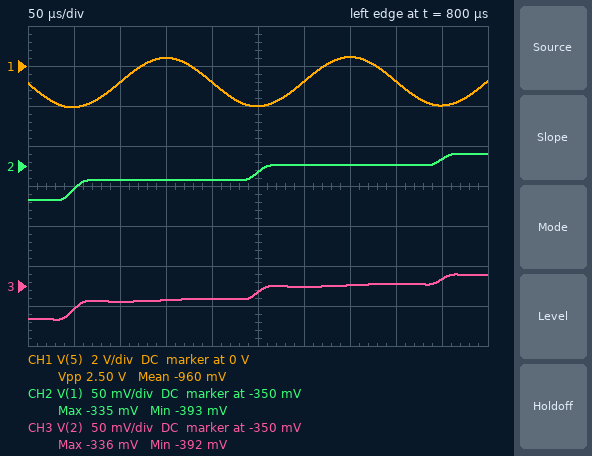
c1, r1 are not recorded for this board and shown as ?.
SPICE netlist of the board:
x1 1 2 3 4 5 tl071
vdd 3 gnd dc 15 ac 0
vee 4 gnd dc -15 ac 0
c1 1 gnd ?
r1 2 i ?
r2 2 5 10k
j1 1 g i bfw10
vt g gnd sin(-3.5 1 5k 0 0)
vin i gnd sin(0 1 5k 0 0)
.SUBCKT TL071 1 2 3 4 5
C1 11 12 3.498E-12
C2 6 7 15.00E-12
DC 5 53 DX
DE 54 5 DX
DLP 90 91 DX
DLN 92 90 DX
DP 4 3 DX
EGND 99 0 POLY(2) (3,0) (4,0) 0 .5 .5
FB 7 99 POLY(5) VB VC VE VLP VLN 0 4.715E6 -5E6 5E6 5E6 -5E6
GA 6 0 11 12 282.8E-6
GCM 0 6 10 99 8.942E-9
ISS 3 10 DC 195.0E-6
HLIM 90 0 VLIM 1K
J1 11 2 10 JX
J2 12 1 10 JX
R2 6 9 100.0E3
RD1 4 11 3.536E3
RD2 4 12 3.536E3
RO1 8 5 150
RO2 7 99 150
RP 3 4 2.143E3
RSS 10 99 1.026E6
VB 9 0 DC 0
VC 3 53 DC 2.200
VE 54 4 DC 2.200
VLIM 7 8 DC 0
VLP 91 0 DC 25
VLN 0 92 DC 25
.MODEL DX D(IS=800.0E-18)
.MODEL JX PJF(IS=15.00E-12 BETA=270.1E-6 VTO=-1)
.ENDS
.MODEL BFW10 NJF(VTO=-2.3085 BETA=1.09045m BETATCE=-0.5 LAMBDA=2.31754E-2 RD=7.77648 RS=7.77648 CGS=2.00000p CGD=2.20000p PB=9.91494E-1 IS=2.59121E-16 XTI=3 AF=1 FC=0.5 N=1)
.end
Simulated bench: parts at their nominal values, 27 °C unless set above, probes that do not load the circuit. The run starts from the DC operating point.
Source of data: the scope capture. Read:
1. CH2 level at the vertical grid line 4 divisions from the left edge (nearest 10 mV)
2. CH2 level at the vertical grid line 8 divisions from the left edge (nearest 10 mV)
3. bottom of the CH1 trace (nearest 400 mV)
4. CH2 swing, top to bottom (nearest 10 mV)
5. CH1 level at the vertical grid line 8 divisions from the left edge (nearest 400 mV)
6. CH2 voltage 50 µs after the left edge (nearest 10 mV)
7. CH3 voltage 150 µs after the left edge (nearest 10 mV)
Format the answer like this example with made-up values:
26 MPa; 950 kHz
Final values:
-370 mV; -350 mV; -2.0 V; 60 mV; -800 mV; -380 mV; -370 mV
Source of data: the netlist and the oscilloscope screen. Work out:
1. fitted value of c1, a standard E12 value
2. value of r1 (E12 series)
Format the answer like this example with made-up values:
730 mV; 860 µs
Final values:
33 nF; 8.2 kΩ
